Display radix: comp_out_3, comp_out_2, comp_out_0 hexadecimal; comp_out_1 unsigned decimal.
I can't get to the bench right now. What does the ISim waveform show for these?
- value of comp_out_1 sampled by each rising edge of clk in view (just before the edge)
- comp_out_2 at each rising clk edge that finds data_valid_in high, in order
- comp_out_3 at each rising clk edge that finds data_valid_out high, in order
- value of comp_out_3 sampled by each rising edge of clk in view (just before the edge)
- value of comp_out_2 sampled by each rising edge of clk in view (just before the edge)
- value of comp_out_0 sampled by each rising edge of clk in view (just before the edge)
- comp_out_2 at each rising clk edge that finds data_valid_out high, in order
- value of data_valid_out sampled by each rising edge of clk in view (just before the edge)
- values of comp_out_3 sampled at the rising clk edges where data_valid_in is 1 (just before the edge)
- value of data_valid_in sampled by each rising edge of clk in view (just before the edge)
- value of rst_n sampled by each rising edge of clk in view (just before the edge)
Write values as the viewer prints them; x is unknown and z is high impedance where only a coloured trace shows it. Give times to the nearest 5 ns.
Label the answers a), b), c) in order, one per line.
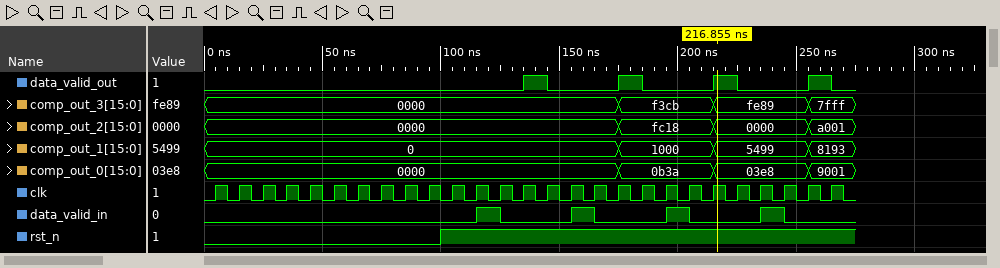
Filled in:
a) 0, 0, 0, 0, 0, 0, 0, 0, 0, 0, 0, 0, 0, 0, 0, 0, 0, 0, 1000, 1000, 1000, 1000, 5499, 5499, 5499, 5499, 8193
b) 0000, 0000, fc18, 0000
c) 0000, f3cb, fe89, 7fff
d) 0000, 0000, 0000, 0000, 0000, 0000, 0000, 0000, 0000, 0000, 0000, 0000, 0000, 0000, 0000, 0000, 0000, 0000, f3cb, f3cb, f3cb, f3cb, fe89, fe89, fe89, fe89, 7fff
e) 0000, 0000, 0000, 0000, 0000, 0000, 0000, 0000, 0000, 0000, 0000, 0000, 0000, 0000, 0000, 0000, 0000, 0000, fc18, fc18, fc18, fc18, 0000, 0000, 0000, 0000, a001
f) 0000, 0000, 0000, 0000, 0000, 0000, 0000, 0000, 0000, 0000, 0000, 0000, 0000, 0000, 0000, 0000, 0000, 0000, 0b3a, 0b3a, 0b3a, 0b3a, 03e8, 03e8, 03e8, 03e8, 9001
g) 0000, fc18, 0000, a001
h) 0 0 0 0 0 0 0 0 0 0 0 0 0 0 1 0 0 0 1 0 0 0 1 0 0 0 1
i) 0000, 0000, f3cb, fe89
j) 0 0 0 0 0 0 0 0 0 0 0 0 1 0 0 0 1 0 0 0 1 0 0 0 1 0 0
k) 0 0 0 0 0 0 0 0 0 0 1 1 1 1 1 1 1 1 1 1 1 1 1 1 1 1 1
